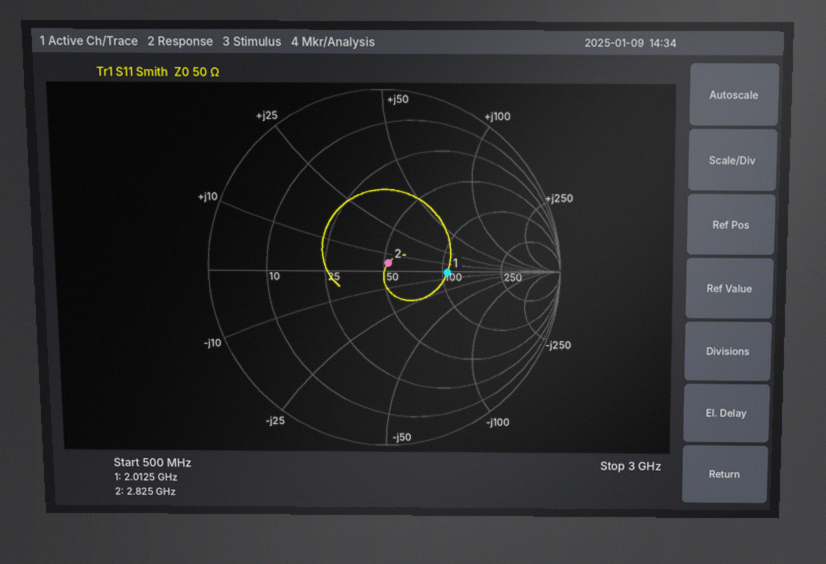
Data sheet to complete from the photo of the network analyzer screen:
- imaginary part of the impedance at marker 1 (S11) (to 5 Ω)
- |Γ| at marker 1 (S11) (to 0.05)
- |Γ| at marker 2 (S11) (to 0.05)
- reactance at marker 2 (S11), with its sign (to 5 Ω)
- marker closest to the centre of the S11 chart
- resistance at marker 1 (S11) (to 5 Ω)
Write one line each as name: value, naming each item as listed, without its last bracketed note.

imaginary part of the impedance at marker 1 (S11): 0 Ω
|Γ| at marker 1 (S11): 0.35
|Γ| at marker 2 (S11): 0.05
reactance at marker 2 (S11), with its sign: +5 Ω
marker closest to the centre of the S11 chart: marker 2
resistance at marker 1 (S11): 105 Ω
